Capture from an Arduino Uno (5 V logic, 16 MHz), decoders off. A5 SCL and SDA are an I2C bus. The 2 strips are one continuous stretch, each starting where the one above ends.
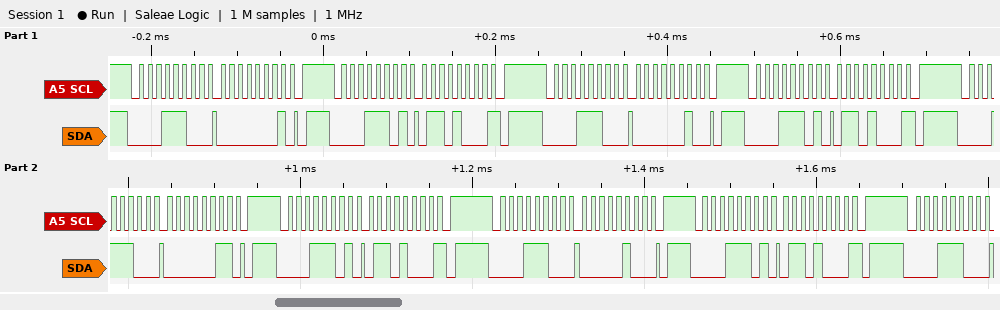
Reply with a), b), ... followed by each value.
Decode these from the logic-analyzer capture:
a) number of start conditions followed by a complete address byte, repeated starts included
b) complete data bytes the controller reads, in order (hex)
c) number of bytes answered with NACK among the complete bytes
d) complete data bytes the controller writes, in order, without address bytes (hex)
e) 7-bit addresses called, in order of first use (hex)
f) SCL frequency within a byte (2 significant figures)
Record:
a) 9
b) 68 68 68 68
c) 4
d) 01 02 03 04
e) 0x0E
f) 100 kHz
